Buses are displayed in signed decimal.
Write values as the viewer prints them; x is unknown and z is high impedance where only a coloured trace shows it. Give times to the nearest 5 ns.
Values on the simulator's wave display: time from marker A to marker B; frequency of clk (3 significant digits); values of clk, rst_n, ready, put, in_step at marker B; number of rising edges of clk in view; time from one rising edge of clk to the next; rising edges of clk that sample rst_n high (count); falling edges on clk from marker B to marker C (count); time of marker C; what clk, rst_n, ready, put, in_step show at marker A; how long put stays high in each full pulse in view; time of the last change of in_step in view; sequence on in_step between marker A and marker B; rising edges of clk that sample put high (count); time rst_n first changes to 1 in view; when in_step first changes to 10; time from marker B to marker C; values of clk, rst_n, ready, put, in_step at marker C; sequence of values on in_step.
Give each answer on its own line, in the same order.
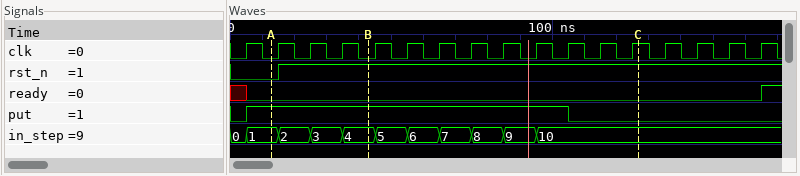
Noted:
30 ns
100 MHz
clk=0, rst_n=1, ready=0, put=1, in_step=4
17
10 ns
15
8
125 ns
clk=0, rst_n=0, ready=0, put=1, in_step=1
100 ns
95 ns
1, 2, 3, 4
10
15 ns
95 ns
85 ns
clk=1, rst_n=1, ready=0, put=0, in_step=10
0, 1, 2, 3, 4, 5, 6, 7, 8, 9, 10
